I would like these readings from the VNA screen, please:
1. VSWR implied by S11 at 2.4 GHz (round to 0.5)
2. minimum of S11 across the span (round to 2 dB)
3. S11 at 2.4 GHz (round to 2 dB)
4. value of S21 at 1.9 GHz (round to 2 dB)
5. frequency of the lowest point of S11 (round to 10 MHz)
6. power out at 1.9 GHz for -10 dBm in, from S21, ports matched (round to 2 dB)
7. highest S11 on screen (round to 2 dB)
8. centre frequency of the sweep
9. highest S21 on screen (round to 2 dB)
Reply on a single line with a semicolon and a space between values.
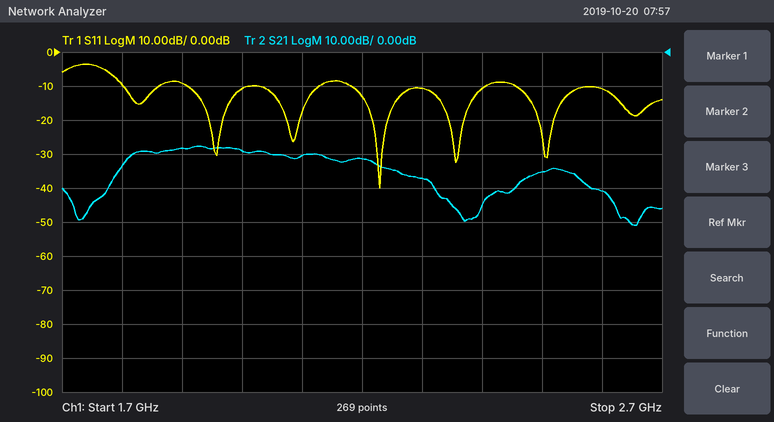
2.0; -40 dB; -10 dB; -28 dB; 2.23 GHz; -38 dBm; -4 dB; 2.2 GHz; -28 dB
